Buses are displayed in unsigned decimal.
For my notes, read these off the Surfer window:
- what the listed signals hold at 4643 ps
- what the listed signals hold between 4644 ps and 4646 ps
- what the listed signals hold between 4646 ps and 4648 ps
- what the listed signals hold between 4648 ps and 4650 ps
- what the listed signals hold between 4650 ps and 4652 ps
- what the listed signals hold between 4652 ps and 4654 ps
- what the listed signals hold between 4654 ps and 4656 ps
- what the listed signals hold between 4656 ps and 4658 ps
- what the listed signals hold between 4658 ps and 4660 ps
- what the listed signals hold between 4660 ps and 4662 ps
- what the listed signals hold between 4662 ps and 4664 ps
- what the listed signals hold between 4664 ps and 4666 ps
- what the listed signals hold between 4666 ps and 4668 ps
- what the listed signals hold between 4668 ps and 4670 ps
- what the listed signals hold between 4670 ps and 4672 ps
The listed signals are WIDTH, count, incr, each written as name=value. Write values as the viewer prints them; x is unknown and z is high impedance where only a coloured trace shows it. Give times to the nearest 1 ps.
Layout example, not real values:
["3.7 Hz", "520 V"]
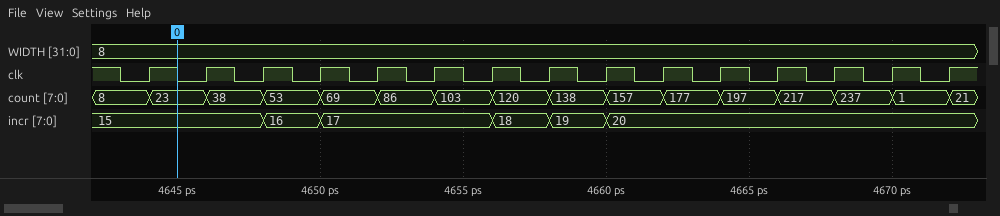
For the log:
["WIDTH=8, count=8, incr=15", "WIDTH=8, count=23, incr=15", "WIDTH=8, count=38, incr=15", "WIDTH=8, count=53, incr=16", "WIDTH=8, count=69, incr=17", "WIDTH=8, count=86, incr=17", "WIDTH=8, count=103, incr=17", "WIDTH=8, count=120, incr=18", "WIDTH=8, count=138, incr=19", "WIDTH=8, count=157, incr=20", "WIDTH=8, count=177, incr=20", "WIDTH=8, count=197, incr=20", "WIDTH=8, count=217, incr=20", "WIDTH=8, count=237, incr=20", "WIDTH=8, count=1, incr=20"]
